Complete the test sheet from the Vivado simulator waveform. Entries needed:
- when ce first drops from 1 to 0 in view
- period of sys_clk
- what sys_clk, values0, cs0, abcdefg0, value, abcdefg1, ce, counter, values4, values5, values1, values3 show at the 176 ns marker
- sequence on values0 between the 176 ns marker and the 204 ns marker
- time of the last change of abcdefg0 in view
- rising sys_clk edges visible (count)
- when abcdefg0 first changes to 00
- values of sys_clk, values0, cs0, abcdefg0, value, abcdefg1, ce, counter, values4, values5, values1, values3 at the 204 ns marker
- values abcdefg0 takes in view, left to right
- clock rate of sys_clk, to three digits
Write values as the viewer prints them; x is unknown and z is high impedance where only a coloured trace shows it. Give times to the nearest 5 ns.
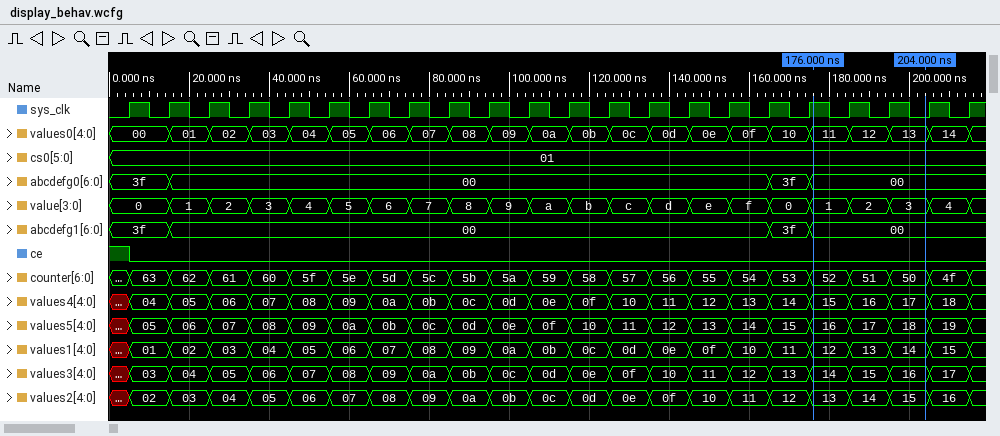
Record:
5 ns
10 ns
sys_clk=1, values0=11, cs0=01, abcdefg0=00, value=1, abcdefg1=00, ce=0, counter=52, values4=15, values5=16, values1=12, values3=14
11, 12, 13
175 ns
22
15 ns
sys_clk=0, values0=13, cs0=01, abcdefg0=00, value=3, abcdefg1=00, ce=0, counter=50, values4=17, values5=18, values1=14, values3=16
3f, 00, 3f, 00
100 MHz
